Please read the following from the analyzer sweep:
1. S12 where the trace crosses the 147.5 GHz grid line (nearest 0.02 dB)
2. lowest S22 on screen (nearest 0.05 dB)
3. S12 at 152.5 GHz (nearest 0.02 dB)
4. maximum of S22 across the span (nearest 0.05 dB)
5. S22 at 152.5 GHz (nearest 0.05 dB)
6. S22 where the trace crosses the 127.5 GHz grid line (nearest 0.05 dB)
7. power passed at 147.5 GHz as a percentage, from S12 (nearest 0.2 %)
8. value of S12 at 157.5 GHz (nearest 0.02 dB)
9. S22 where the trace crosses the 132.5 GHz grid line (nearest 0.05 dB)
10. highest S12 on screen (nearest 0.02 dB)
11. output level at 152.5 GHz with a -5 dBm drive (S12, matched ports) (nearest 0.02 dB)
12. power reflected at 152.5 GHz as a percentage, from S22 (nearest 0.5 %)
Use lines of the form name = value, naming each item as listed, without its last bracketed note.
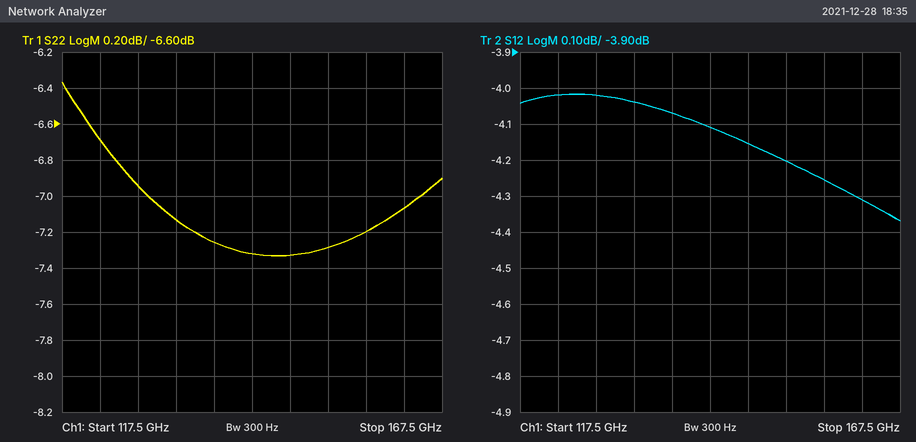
S12 where the trace crosses the 147.5 GHz grid line = -4.16 dB
lowest S22 on screen = -7.35 dB
S12 at 152.5 GHz = -4.20 dB
maximum of S22 across the span = -6.35 dB
S22 at 152.5 GHz = -7.30 dB
S22 where the trace crosses the 127.5 GHz grid line = -6.95 dB
power passed at 147.5 GHz as a percentage, from S12 = 38.4 %
value of S12 at 157.5 GHz = -4.26 dB
S22 where the trace crosses the 132.5 GHz grid line = -7.15 dB
highest S12 on screen = -4.02 dB
output level at 152.5 GHz with a -5 dBm drive (S12, matched ports) = -9.20 dBm
power reflected at 152.5 GHz as a percentage, from S22 = 18.5 %
